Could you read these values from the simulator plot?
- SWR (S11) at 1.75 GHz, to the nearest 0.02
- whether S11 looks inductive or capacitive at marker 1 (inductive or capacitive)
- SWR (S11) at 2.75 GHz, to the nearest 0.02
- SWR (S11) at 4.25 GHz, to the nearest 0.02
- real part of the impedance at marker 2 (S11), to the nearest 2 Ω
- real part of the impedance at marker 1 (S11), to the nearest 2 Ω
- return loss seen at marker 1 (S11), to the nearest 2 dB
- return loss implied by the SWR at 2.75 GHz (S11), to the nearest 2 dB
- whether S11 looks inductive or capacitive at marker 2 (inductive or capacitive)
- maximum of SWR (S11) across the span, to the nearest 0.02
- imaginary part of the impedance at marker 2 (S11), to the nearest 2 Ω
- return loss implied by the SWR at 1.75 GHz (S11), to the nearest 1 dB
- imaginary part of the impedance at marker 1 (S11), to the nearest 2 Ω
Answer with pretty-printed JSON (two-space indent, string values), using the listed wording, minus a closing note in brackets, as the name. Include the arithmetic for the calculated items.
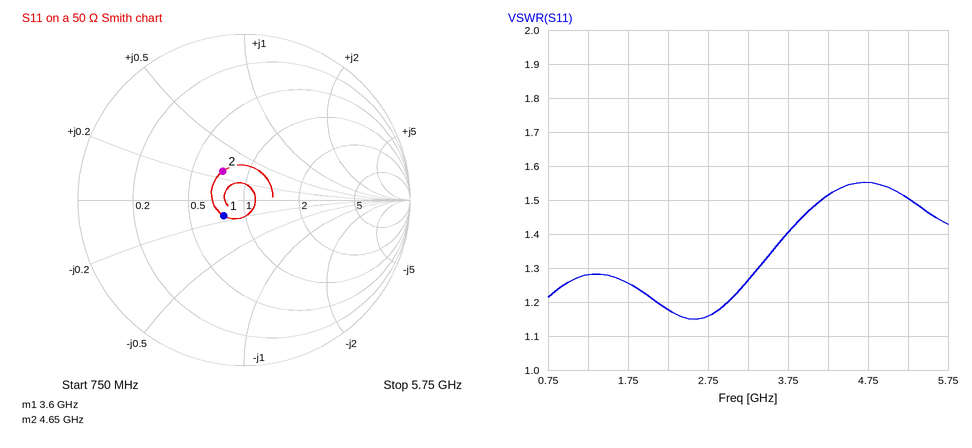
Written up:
{
  "SWR (S11) at 1.75 GHz, to the nearest 0.02": "1.26",
  "whether S11 looks inductive or capacitive at marker 1": "capacitive",
  "SWR (S11) at 2.75 GHz, to the nearest 0.02": "1.16",
  "SWR (S11) at 4.25 GHz, to the nearest 0.02": "1.52",
  "real part of the impedance at marker 2 (S11), to the nearest 2 Ω": "36 Ω",
  "real part of the impedance at marker 1 (S11), to the nearest 2 Ω": "38 Ω",
  "return loss seen at marker 1 (S11), to the nearest 2 dB": "16 dB",
  "return loss implied by the SWR at 2.75 GHz (S11), to the nearest 2 dB": "−20 log10((1.16 − 1)/(1.16 + 1)) ≈ 22.6 dB, so 22 dB to the nearest 2 dB",
  "whether S11 looks inductive or capacitive at marker 2": "inductive",
  "maximum of SWR (S11) across the span, to the nearest 0.02": "1.56",
  "imaginary part of the impedance at marker 2 (S11), to the nearest 2 Ω": "+14 Ω",
  "return loss implied by the SWR at 1.75 GHz (S11), to the nearest 1 dB": "−20 log10((1.26 − 1)/(1.26 + 1)) ≈ 19 dB",
  "imaginary part of the impedance at marker 1 (S11), to the nearest 2 Ω": "-8 Ω"
}
